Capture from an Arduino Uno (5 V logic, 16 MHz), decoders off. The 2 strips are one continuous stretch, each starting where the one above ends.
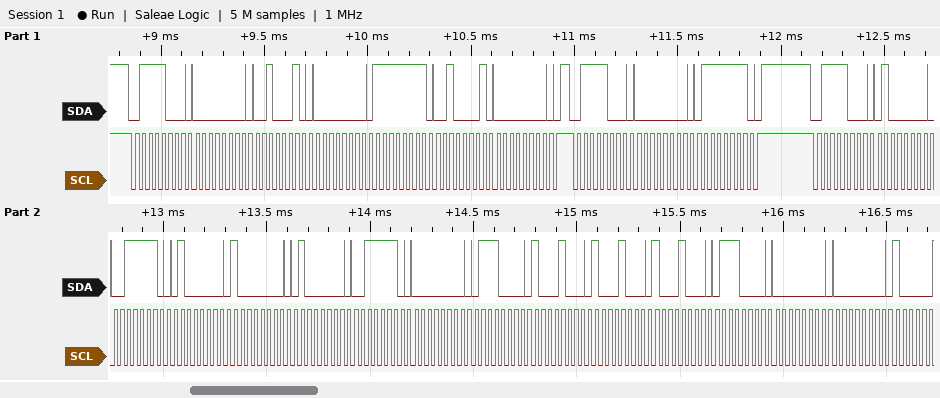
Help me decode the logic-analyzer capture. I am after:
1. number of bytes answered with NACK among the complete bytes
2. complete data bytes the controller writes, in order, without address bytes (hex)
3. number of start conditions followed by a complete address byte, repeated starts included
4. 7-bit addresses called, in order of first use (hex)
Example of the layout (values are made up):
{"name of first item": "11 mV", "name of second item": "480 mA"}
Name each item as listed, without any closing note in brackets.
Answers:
{"number of bytes answered with NACK among the complete bytes": "0", "complete data bytes the controller writes, in order, without address bytes": "00 22 00 FF 21 00 00 7F 40 3E 40 80 40 3E 00 70 88 88 88 70 00 00", "number of start conditions followed by a complete address byte, repeated starts included": "3", "7-bit addresses called, in order of first use": "0x3C"}
